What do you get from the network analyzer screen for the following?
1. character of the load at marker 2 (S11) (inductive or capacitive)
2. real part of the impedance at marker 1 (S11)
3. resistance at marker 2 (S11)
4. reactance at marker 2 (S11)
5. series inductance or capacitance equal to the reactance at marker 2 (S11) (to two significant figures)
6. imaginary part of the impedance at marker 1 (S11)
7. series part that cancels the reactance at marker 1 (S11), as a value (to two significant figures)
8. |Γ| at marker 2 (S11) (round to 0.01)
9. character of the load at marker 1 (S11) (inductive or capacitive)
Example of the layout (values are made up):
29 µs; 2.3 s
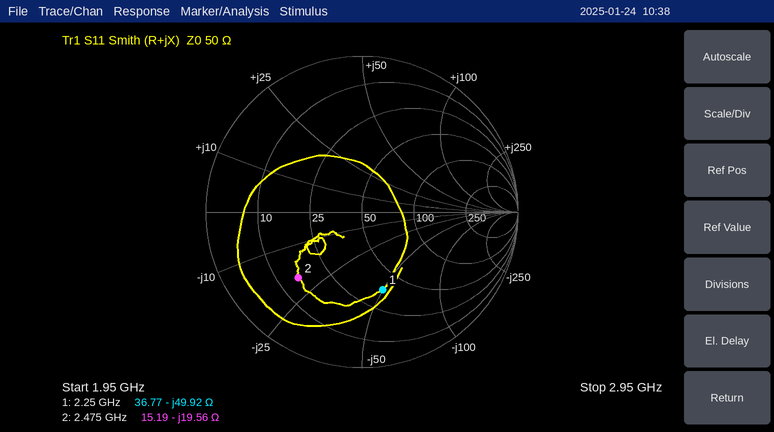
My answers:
capacitive; 36.77 Ω; 15.19 Ω; -19.56 Ω; 3.3 pF; -49.92 Ω; 3.5 nH; 0.59; capacitive
